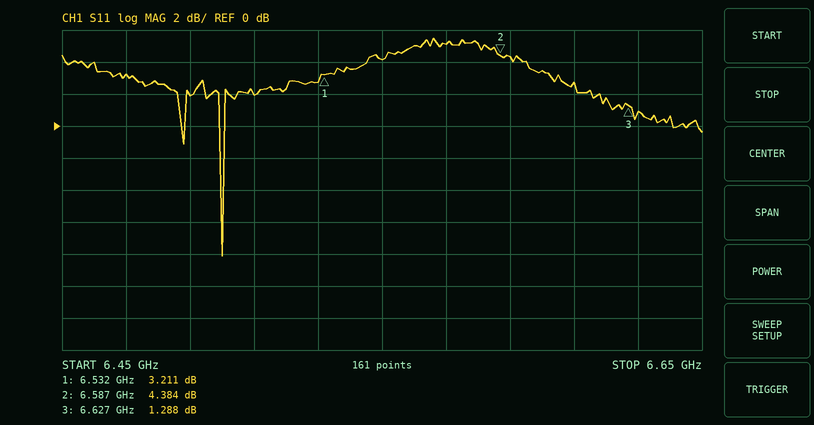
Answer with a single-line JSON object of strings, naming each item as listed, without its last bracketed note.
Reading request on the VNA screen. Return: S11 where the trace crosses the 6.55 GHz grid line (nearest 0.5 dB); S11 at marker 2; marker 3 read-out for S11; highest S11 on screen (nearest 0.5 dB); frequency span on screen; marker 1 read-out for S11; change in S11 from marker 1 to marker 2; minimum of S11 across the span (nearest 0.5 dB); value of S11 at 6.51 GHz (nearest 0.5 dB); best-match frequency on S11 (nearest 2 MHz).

{"S11 where the trace crosses the 6.55 GHz grid line": "4.0 dB", "S11 at marker 2": "4.384 dB", "marker 3 read-out for S11": "1.288 dB", "highest S11 on screen": "5.5 dB", "frequency span on screen": "200 MHz", "marker 1 read-out for S11": "3.211 dB", "change in S11 from marker 1 to marker 2": "1.173 dB", "minimum of S11 across the span": "-8.0 dB", "value of S11 at 6.51 GHz": "2.0 dB", "best-match frequency on S11": "6.500 GHz"}
